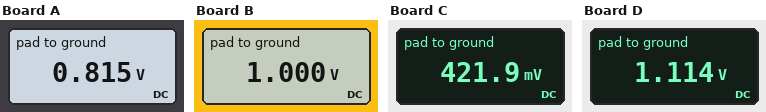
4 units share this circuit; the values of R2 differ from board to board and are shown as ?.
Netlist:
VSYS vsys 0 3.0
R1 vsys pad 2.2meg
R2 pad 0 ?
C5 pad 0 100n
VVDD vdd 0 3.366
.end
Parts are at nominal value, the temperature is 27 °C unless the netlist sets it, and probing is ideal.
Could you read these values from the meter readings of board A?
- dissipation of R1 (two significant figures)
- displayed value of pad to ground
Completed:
2.2 µW
0.815 V
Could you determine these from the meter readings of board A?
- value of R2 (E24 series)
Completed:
820 kΩ
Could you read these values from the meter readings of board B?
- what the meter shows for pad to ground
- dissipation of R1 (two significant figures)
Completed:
1.000 V
1.8 µW
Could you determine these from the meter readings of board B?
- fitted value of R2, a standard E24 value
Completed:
1.1 MΩ
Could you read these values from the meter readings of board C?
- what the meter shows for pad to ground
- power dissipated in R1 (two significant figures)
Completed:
421.9 mV
3.0 µW
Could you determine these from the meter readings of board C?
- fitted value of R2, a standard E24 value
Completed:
360 kΩ
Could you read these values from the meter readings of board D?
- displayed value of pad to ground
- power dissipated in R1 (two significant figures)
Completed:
1.114 V
1.6 µW
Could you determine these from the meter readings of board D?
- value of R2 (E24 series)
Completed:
1.3 MΩ
